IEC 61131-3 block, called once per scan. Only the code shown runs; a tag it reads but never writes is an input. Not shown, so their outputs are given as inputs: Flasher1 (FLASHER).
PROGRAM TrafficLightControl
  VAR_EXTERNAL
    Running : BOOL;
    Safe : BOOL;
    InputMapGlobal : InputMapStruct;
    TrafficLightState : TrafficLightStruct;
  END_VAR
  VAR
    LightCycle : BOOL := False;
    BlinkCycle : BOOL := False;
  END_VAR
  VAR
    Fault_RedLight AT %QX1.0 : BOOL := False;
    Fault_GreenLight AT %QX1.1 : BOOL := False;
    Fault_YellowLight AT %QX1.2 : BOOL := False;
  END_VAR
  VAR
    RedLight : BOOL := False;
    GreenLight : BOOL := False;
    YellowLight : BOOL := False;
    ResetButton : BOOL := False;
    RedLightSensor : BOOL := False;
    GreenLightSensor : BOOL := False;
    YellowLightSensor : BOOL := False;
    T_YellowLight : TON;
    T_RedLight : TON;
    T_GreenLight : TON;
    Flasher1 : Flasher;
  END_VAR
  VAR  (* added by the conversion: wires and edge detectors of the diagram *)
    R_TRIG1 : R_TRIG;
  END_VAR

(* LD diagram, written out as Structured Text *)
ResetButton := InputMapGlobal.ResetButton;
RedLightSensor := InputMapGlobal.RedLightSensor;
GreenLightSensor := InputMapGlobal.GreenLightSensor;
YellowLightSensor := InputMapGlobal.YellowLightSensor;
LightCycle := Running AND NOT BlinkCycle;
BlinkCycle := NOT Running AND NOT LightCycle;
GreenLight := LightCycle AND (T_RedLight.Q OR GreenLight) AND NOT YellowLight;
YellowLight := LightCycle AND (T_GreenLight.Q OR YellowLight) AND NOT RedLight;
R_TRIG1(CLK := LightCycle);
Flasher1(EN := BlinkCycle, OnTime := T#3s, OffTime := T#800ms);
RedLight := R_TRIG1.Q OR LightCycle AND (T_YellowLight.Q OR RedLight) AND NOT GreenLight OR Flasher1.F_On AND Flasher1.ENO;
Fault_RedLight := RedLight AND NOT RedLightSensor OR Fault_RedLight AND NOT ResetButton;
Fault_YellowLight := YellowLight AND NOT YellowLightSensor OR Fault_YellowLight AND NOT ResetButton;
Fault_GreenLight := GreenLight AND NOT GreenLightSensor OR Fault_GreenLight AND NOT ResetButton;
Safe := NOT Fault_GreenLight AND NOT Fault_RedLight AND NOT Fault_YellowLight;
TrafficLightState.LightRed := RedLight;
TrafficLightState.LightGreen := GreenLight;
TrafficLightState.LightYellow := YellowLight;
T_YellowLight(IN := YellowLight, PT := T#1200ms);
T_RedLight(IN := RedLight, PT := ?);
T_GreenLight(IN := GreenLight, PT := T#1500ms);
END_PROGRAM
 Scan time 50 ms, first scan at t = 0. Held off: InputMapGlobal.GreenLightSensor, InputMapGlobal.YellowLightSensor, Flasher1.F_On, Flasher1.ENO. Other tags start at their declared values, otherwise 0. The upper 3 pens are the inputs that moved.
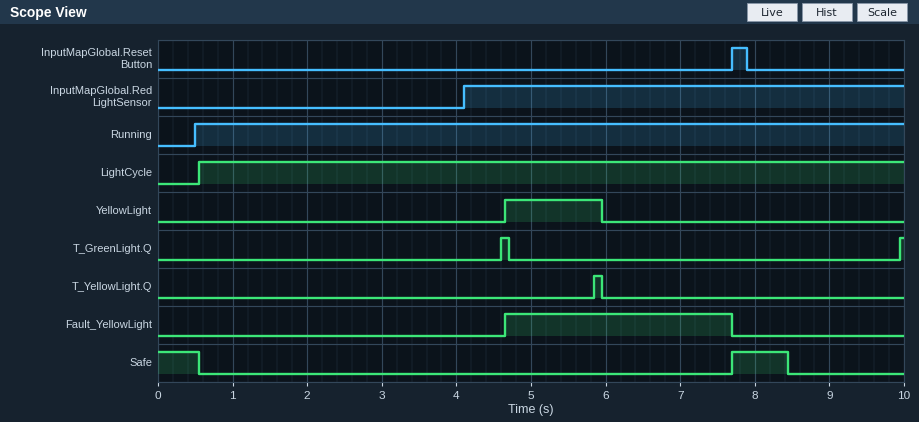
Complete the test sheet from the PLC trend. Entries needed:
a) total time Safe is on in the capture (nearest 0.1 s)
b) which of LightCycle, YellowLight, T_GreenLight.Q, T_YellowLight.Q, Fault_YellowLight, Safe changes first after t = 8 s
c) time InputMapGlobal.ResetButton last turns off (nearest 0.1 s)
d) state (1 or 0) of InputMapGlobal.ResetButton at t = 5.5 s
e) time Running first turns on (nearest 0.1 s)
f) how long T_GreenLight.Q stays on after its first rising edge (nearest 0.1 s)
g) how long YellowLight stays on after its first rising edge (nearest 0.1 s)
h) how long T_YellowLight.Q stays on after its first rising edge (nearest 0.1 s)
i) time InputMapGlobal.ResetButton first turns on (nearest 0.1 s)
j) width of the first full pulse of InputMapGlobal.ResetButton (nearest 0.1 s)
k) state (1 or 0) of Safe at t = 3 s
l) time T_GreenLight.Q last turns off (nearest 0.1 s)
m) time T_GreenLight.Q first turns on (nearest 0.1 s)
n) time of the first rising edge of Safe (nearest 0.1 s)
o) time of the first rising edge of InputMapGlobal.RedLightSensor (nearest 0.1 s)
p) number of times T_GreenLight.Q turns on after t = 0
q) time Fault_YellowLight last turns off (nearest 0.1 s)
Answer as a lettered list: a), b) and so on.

a) 1.3 s
b) Safe
c) 7.9 s
d) 0
e) 0.5 s
f) 0.1 s
g) 1.3 s
h) 0.1 s
i) 7.7 s
j) 0.2 s
k) 0
l) 4.7 s
m) 4.6 s
n) 7.7 s
o) 4.1 s
p) 2
q) 7.7 s
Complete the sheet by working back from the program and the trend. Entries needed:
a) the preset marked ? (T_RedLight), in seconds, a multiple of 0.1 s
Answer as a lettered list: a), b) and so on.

a) 2.5 s
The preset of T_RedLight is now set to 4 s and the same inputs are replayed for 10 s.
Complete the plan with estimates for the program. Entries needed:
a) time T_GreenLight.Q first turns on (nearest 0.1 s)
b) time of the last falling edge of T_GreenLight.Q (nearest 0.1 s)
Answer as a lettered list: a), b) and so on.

a) 6.1 s
b) 6.2 s
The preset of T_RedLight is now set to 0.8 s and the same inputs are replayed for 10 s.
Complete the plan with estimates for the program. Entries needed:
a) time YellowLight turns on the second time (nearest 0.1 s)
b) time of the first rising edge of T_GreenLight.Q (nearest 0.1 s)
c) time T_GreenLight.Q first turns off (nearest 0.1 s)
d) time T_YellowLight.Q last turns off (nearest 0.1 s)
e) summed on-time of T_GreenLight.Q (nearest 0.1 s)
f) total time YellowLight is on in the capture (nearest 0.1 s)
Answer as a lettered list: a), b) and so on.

a) 6.6 s
b) 2.9 s
c) 3.0 s
d) 7.9 s
e) 0.2 s
f) 2.6 s
